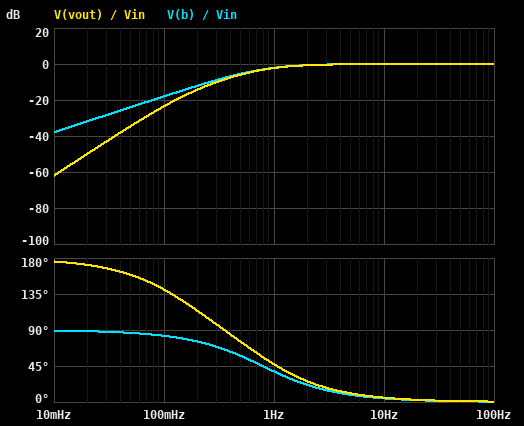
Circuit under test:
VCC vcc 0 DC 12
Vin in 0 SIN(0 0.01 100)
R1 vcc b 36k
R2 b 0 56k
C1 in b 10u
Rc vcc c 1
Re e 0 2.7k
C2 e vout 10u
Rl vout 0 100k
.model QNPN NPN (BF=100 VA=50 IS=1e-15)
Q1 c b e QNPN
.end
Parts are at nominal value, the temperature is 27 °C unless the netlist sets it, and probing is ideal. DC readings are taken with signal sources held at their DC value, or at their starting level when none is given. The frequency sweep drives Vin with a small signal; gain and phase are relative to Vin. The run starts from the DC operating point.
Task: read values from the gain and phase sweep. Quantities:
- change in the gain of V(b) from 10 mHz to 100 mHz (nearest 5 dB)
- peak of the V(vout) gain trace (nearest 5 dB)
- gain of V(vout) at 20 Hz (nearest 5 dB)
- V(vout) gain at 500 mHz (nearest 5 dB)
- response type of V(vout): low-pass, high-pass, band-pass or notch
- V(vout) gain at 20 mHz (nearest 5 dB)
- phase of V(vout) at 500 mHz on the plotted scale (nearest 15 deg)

20 dB
0 dB
0 dB
-5 dB
high-pass
-50 dB
75 deg
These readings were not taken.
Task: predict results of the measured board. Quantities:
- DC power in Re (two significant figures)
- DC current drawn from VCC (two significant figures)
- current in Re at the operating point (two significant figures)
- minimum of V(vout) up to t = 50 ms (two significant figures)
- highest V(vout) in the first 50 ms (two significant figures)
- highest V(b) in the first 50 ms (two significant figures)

14 mW
2.4 mA
2.3 mA
-10 mV
9.9 mV
6.9 V
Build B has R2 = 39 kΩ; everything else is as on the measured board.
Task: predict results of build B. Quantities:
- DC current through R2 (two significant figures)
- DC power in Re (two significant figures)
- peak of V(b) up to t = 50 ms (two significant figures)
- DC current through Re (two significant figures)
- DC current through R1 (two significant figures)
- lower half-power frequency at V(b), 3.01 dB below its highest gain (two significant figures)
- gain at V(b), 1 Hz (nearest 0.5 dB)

150 µA
10 mW
5.9 V
1.9 mA
170 µA
910 mHz
-2.5 dB
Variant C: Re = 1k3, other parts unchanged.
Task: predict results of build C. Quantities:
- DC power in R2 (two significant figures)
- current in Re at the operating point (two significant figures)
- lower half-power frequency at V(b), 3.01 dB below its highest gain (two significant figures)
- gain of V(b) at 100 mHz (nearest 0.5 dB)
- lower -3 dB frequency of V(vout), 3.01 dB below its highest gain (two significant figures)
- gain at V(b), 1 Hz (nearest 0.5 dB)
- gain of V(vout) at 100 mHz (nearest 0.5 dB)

740 µW
4.4 mA
850 mHz
-18.5 dB
880 mHz
-2.5 dB
-24.0 dB
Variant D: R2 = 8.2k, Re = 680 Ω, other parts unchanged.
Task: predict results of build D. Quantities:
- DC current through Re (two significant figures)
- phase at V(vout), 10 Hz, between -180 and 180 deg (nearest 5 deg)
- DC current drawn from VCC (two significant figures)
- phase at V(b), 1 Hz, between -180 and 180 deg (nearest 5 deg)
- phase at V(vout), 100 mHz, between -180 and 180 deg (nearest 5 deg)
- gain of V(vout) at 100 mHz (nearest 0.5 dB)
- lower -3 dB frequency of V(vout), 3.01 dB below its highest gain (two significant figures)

2.0 mA
15 deg
2.3 mA
70 deg
145 deg
-34.0 dB
2.6 Hz
